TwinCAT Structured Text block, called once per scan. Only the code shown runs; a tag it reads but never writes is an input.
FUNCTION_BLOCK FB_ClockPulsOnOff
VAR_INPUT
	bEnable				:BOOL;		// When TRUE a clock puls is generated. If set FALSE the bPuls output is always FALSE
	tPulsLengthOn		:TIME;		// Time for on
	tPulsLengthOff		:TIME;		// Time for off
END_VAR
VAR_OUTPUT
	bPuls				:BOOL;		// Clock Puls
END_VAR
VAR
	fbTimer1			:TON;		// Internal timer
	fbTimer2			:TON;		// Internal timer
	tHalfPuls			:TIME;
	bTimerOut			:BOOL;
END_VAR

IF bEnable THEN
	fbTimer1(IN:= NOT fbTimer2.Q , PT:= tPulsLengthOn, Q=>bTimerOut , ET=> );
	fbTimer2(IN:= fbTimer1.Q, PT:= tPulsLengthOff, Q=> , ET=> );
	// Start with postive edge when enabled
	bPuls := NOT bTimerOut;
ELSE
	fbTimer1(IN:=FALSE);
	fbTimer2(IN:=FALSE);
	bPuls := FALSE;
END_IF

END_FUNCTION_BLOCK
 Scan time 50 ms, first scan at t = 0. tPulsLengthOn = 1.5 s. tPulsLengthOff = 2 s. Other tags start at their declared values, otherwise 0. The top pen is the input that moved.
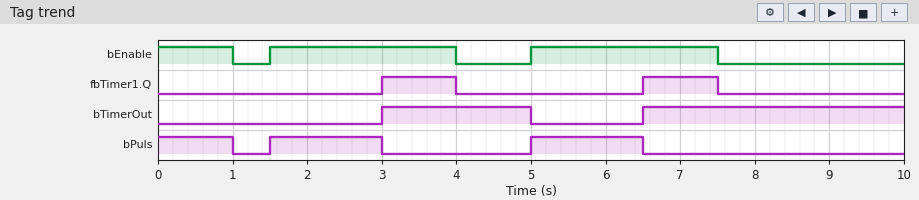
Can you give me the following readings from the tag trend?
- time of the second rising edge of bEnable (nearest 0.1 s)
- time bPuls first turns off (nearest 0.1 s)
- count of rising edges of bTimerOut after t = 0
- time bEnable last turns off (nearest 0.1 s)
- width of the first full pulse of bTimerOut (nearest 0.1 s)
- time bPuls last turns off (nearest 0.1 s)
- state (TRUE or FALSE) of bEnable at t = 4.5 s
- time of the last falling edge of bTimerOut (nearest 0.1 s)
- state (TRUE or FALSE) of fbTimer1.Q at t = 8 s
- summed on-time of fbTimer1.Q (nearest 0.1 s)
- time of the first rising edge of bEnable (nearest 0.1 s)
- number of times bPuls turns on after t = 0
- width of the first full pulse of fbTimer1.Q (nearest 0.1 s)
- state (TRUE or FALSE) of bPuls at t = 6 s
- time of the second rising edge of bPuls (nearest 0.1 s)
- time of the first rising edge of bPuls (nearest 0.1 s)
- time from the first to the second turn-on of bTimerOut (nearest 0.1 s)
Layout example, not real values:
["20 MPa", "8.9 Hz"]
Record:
["5.0 s", "1.0 s", "2", "7.5 s", "2.0 s", "6.5 s", "FALSE", "5.0 s", "FALSE", "2.0 s", "1.5 s", "2", "1.0 s", "TRUE", "5.0 s", "1.5 s", "3.5 s"]
